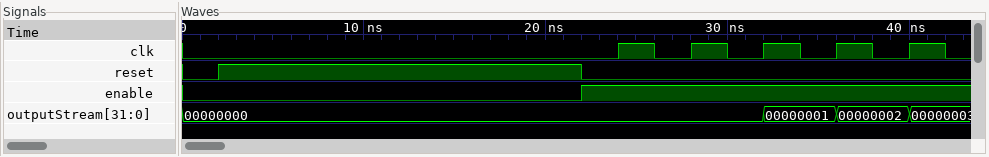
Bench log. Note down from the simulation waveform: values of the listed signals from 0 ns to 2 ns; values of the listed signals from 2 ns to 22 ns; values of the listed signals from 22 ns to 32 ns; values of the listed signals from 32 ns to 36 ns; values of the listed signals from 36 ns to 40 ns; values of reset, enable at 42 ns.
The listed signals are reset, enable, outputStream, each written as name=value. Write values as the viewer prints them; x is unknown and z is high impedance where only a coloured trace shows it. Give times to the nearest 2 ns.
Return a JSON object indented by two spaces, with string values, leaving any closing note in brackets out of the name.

{
  "values of the listed signals from 0 ns to 2 ns": "reset=0, enable=0, outputStream=00000000",
  "values of the listed signals from 2 ns to 22 ns": "reset=1, enable=0, outputStream=00000000",
  "values of the listed signals from 22 ns to 32 ns": "reset=0, enable=1, outputStream=00000000",
  "values of the listed signals from 32 ns to 36 ns": "reset=0, enable=1, outputStream=00000001",
  "values of the listed signals from 36 ns to 40 ns": "reset=0, enable=1, outputStream=00000002",
  "values of reset, enable at 42 ns": "reset=0, enable=1"
}
